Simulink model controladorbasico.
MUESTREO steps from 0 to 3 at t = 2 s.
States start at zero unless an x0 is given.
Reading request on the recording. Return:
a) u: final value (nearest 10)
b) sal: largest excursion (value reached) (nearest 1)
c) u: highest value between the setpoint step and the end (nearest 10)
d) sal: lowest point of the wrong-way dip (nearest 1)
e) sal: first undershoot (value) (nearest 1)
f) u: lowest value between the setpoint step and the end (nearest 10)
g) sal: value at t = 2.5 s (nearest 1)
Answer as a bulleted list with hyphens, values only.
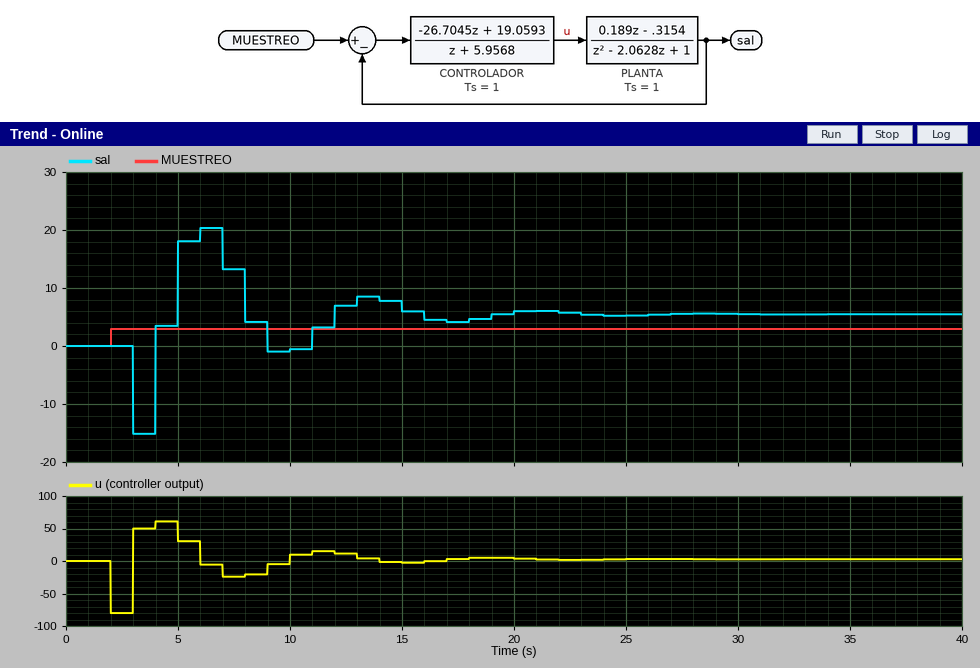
- 0
- 20
- 60
- -15
- -1
- -80
- 0
